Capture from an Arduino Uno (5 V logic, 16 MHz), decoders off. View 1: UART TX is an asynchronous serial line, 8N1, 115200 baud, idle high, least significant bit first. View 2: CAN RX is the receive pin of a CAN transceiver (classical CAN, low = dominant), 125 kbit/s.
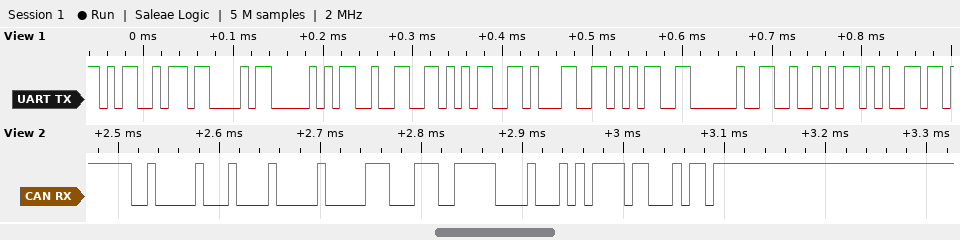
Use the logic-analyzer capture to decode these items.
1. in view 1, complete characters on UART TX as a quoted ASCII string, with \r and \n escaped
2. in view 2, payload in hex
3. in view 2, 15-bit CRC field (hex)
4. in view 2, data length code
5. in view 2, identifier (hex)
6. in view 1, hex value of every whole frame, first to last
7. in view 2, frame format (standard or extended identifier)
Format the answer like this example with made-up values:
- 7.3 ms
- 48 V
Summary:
- "MCP2515 Re"
- 00 C7 3E 22
- 0x5EC5
- 4
- 0x201
- 0x4D 0x43 0x50 0x32 0x35 0x31 0x35 0x20 0x52 0x65
- standard
